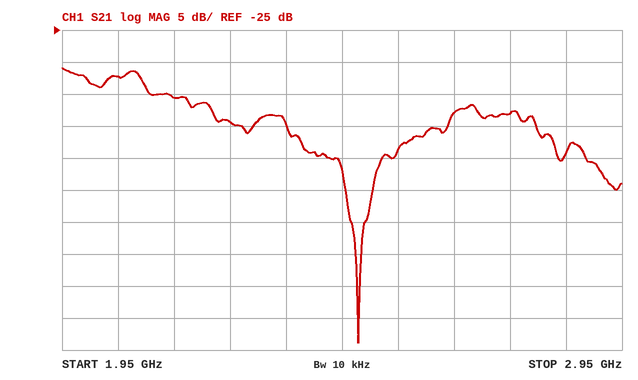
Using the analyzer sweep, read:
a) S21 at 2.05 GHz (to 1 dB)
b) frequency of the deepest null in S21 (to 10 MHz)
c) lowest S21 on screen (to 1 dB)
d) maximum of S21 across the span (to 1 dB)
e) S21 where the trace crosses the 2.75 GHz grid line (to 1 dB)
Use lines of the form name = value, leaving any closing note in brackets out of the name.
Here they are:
S21 at 2.05 GHz = -32 dB
frequency of the deepest null in S21 = 2.48 GHz
lowest S21 on screen = -74 dB
maximum of S21 across the span = -31 dB
S21 where the trace crosses the 2.75 GHz grid line = -38 dB
